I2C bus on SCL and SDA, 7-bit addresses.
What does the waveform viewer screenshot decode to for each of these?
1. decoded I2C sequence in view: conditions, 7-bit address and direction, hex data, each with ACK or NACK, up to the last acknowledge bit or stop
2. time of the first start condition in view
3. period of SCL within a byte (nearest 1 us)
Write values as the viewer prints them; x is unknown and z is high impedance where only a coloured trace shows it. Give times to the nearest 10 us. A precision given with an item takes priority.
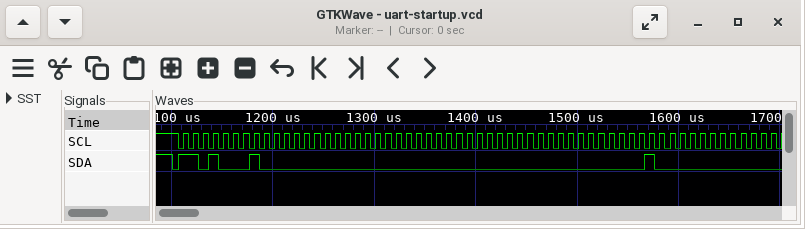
start, address 68 read ACK, 00 ACK, 00 ACK, 00 ACK, 00 ACK, 40 ACK
1100 us
10 us
